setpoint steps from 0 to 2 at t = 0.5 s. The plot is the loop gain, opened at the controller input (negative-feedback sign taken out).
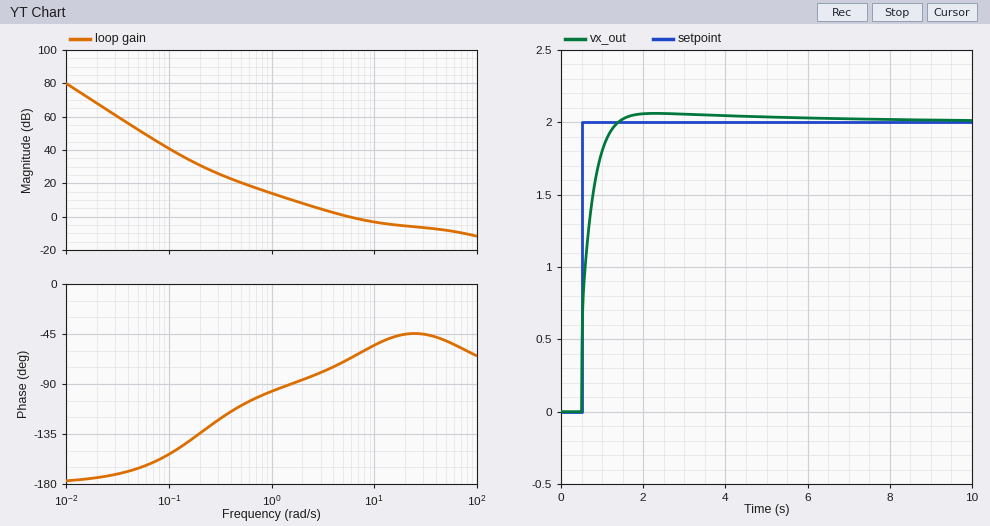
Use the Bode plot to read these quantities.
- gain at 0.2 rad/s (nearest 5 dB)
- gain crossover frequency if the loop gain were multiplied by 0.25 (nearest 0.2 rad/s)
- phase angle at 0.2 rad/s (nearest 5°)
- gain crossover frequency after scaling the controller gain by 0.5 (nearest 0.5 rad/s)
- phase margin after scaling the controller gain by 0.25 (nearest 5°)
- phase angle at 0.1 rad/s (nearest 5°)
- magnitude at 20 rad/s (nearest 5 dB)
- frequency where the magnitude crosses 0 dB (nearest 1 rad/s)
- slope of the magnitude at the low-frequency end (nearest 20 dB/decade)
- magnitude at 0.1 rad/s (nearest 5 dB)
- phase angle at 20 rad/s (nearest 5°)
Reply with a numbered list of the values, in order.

1. 30 dB
2. 1.2 rad/s
3. -135°
4. 2.5 rad/s
5. 85°
6. -155°
7. -5 dB
8. 6 rad/s
9. -40 dB/decade
10. 40 dB
11. -45°
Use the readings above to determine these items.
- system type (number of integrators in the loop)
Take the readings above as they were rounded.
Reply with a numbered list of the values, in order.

1. 2
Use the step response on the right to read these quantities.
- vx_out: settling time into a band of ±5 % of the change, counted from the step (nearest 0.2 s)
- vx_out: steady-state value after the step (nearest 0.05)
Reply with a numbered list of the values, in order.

1. 0.6 s
2. 2.00
